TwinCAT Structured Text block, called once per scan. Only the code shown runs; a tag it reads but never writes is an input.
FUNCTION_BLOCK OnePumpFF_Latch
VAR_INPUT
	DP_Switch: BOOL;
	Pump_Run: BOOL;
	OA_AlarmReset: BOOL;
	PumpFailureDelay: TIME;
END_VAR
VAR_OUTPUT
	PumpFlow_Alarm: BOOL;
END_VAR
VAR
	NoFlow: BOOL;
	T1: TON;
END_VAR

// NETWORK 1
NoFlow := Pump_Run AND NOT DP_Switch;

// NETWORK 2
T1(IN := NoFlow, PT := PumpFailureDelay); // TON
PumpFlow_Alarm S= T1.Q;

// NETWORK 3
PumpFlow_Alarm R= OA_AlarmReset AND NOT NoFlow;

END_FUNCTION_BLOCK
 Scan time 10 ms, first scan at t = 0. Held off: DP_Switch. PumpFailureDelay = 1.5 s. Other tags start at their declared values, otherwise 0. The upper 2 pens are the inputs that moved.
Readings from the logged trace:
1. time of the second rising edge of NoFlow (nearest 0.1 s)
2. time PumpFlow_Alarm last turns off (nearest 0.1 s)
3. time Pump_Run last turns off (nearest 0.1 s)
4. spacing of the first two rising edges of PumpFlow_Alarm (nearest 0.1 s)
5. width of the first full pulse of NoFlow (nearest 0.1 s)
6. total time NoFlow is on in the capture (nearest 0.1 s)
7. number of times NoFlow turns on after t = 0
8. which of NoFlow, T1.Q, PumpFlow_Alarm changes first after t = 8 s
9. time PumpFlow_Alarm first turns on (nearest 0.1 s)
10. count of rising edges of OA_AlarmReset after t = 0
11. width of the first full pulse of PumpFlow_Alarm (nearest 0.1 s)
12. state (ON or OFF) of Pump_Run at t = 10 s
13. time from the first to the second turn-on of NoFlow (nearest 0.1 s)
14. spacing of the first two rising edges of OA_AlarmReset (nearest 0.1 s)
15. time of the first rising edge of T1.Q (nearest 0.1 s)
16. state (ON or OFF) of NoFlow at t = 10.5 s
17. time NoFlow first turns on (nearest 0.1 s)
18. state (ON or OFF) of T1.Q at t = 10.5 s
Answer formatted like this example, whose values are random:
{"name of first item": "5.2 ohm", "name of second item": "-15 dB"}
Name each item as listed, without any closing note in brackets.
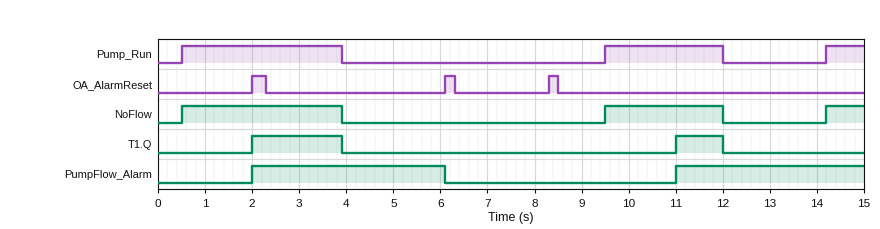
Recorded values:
{"time of the second rising edge of NoFlow": "9.5 s", "time PumpFlow_Alarm last turns off": "6.1 s", "time Pump_Run last turns off": "12.0 s", "spacing of the first two rising edges of PumpFlow_Alarm": "9.0 s", "width of the first full pulse of NoFlow": "3.4 s", "total time NoFlow is on in the capture": "6.7 s", "number of times NoFlow turns on after t = 0": "3", "which of NoFlow, T1.Q, PumpFlow_Alarm changes first after t = 8 s": "NoFlow", "time PumpFlow_Alarm first turns on": "2.0 s", "count of rising edges of OA_AlarmReset after t = 0": "3", "width of the first full pulse of PumpFlow_Alarm": "4.1 s", "state (ON or OFF) of Pump_Run at t = 10 s": "ON", "time from the first to the second turn-on of NoFlow": "9.0 s", "spacing of the first two rising edges of OA_AlarmReset": "4.1 s", "time of the first rising edge of T1.Q": "2.0 s", "state (ON or OFF) of NoFlow at t = 10.5 s": "ON", "time NoFlow first turns on": "0.5 s", "state (ON or OFF) of T1.Q at t = 10.5 s": "OFF"}
